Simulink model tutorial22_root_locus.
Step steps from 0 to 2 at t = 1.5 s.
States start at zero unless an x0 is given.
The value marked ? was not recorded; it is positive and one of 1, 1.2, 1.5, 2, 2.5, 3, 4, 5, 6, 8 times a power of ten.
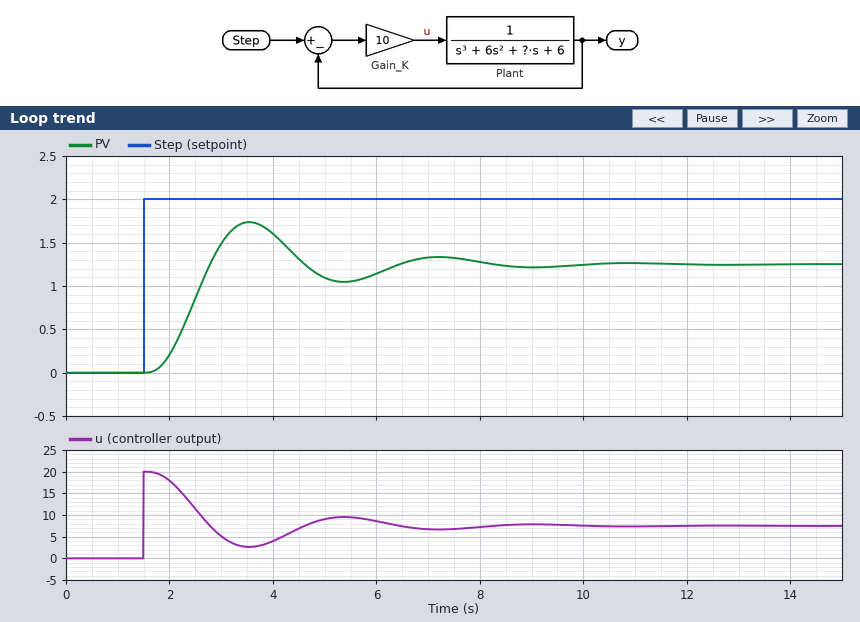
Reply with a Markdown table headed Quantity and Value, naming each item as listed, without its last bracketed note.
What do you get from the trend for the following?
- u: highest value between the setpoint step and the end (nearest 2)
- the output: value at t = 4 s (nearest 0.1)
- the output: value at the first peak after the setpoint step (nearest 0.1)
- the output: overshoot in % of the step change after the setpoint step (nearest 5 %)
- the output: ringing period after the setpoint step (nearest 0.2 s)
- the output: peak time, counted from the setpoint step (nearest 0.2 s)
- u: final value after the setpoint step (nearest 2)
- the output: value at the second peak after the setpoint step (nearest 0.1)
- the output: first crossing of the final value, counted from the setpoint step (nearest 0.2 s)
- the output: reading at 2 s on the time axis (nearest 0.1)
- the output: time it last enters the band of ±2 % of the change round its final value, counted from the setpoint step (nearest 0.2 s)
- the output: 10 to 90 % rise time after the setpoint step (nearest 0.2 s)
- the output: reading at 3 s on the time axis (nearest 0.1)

| Quantity | Value |
|---|---|
| u: highest value between the setpoint step and the end | 20 |
| the output: value at t = 4 s | 1.6 |
| the output: value at the first peak after the setpoint step | 1.7 |
| the output: overshoot in % of the step change after the setpoint step | 40 % |
| the output: ringing period after the setpoint step | 3.6 s |
| the output: peak time, counted from the setpoint step | 2.0 s |
| u: final value after the setpoint step | 8 |
| the output: value at the second peak after the setpoint step | 1.3 |
| the output: first crossing of the final value, counted from the setpoint step | 1.2 s |
| the output: reading at 2 s on the time axis | 0.2 |
| the output: time it last enters the band of ±2 % of the change round its final value, counted from the setpoint step | 8.0 s |
| the output: 10 to 90 % rise time after the setpoint step | 0.8 s |
| the output: reading at 3 s on the time axis | 1.5 |
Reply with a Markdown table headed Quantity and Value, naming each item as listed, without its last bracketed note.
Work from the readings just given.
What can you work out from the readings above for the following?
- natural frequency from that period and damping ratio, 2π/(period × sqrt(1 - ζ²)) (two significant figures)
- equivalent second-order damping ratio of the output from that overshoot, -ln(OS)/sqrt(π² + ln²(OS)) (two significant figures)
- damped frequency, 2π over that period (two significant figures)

| Quantity | Value |
|---|---|
| natural frequency from that period and damping ratio, 2π/(period × sqrt(1 - ζ²)) | 1.8 rad/s |
| equivalent second-order damping ratio of the output from that overshoot, -ln(OS)/sqrt(π² + ln²(OS)) | 0.28 |
| damped frequency, 2π over that period | 1.7 rad/s |
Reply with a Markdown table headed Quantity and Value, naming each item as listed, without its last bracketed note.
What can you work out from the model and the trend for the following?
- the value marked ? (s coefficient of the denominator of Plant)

| Quantity | Value |
|---|---|
| the value marked ? | 8 |
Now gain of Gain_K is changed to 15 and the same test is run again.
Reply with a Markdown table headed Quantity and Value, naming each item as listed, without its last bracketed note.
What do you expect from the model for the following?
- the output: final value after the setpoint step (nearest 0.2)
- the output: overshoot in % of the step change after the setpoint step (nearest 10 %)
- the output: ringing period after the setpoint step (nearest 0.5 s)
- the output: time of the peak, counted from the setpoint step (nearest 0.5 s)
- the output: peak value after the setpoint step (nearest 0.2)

| Quantity | Value |
|---|---|
| the output: final value after the setpoint step | 1.4 |
| the output: overshoot in % of the step change after the setpoint step | 50 % |
| the output: ringing period after the setpoint step | 3.0 s |
| the output: time of the peak, counted from the setpoint step | 2.0 s |
| the output: peak value after the setpoint step | 2.2 |
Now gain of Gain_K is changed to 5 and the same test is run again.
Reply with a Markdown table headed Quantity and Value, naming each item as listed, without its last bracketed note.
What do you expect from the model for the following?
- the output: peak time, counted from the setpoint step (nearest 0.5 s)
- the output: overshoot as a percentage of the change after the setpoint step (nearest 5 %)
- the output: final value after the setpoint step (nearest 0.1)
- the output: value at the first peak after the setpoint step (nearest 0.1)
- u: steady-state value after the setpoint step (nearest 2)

| Quantity | Value |
|---|---|
| the output: peak time, counted from the setpoint step | 2.5 s |
| the output: overshoot as a percentage of the change after the setpoint step | 25 % |
| the output: final value after the setpoint step | 0.9 |
| the output: value at the first peak after the setpoint step | 1.1 |
| u: steady-state value after the setpoint step | 6 |
